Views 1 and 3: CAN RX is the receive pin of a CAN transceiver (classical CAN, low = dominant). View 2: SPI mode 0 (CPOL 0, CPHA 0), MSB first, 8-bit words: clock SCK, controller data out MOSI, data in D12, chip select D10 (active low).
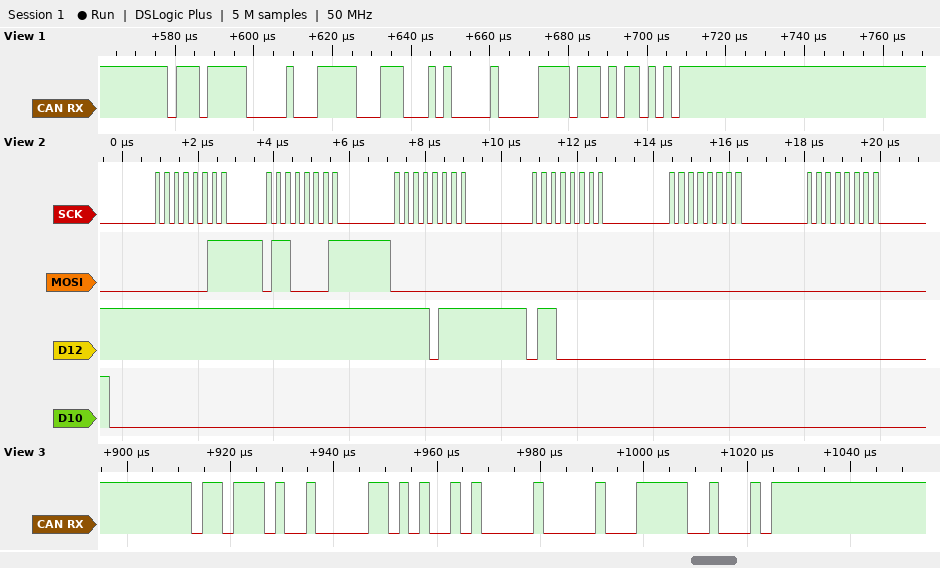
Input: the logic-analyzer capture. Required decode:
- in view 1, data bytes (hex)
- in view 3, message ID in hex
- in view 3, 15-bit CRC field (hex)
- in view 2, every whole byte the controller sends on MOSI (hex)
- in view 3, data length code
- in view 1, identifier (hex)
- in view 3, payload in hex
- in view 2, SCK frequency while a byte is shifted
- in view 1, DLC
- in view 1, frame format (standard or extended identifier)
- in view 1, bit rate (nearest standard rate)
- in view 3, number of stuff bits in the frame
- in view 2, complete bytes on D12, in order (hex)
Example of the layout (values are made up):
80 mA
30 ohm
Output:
E7 14 00
0x6E9
0x03E8
03 61 00 00 00 00
2
0x77C
A5 00
4 MHz
3
standard
500 kbit/s
4
FF FF F7 60 00 00
